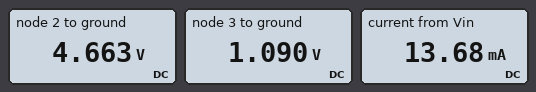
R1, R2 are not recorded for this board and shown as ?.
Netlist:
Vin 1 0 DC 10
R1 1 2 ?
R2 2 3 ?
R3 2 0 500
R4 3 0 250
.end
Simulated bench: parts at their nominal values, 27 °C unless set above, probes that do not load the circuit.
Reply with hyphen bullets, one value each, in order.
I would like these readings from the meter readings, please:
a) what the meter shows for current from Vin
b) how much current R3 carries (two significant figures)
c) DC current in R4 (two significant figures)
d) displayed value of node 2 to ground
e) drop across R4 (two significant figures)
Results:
- 13.68 mA
- 9.3 mA
- 4.4 mA
- 4.663 V
- 1.1 V
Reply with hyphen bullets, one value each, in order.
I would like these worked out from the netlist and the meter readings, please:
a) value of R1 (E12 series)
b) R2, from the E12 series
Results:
- 390 Ω
- 820 Ω
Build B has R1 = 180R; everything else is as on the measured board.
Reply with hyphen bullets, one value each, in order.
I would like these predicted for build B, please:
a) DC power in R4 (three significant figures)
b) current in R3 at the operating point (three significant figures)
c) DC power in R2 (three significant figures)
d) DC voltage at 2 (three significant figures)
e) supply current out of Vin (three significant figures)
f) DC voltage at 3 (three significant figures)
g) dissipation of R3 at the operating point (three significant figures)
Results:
- 9.35 mW
- 13.1 mA
- 30.7 mW
- 6.54 V
- 19.2 mA
- 1.53 V
- 85.6 mW
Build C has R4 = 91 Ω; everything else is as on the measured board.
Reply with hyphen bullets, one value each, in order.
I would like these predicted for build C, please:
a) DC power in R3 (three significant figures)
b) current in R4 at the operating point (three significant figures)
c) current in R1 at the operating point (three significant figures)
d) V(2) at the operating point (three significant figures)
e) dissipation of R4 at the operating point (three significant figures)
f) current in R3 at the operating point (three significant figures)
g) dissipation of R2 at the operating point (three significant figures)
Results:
- 41.0 mW
- 4.97 mA
- 14.0 mA
- 4.53 V
- 2.25 mW
- 9.06 mA
- 20.3 mW
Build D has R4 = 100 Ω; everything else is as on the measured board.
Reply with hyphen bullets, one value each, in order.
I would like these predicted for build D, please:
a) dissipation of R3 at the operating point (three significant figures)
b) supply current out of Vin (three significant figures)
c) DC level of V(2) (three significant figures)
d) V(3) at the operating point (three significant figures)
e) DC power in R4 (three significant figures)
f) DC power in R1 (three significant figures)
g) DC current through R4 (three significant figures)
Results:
- 41.2 mW
- 14.0 mA
- 4.54 V
- 493 mV
- 2.43 mW
- 76.5 mW
- 4.93 mA
